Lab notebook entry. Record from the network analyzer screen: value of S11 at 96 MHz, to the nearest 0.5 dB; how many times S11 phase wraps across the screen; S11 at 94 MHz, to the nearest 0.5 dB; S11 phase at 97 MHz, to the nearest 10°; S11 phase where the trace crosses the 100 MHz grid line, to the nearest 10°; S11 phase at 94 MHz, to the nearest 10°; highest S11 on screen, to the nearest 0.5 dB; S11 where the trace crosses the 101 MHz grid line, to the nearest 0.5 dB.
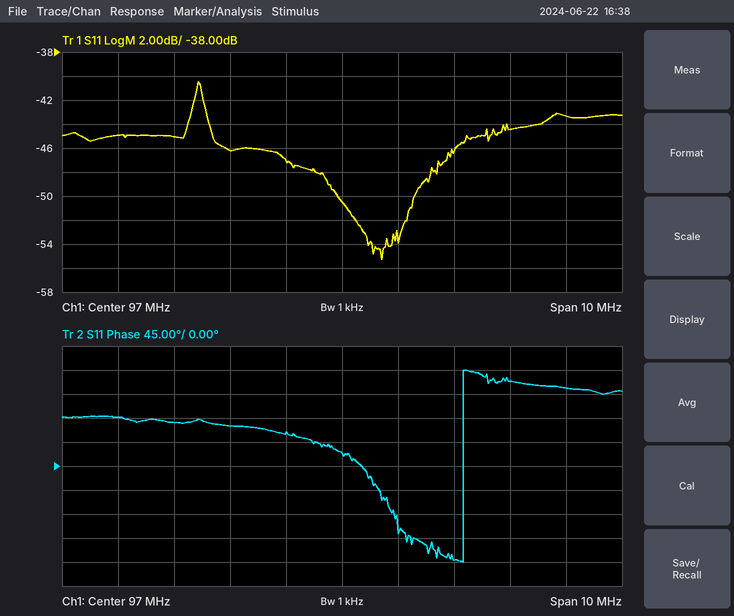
-47.0 dB
1
-45.0 dB
20°
160°
80°
-40.5 dB
-43.5 dB
